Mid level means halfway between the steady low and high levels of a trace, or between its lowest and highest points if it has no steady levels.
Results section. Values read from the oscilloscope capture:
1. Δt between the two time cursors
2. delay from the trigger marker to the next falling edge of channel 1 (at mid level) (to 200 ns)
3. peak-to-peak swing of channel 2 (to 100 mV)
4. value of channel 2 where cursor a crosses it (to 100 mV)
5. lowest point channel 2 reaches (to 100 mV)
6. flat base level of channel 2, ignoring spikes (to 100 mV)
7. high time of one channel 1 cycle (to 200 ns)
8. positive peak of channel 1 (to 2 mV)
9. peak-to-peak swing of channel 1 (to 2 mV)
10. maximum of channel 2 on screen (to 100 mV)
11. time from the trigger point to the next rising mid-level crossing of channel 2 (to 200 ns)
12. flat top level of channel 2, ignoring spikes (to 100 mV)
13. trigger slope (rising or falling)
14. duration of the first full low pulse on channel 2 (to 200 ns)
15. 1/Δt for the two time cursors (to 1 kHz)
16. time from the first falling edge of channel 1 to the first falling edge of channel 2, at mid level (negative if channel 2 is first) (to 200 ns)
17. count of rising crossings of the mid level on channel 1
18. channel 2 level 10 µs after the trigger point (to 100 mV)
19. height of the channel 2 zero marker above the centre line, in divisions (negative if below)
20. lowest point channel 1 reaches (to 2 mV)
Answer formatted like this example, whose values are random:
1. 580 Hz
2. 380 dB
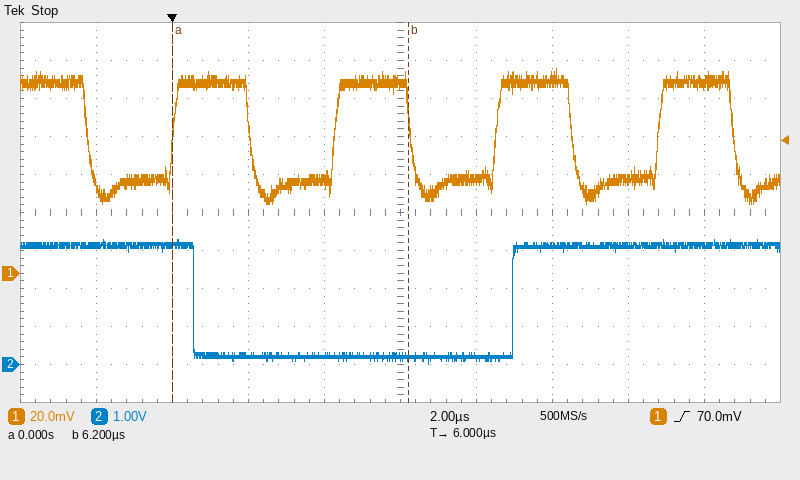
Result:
1. 6.2 µs
2. 2.0 µs
3. 3.3 V
4. 3.1 V
5. 0.0 V
6. 200 mV
7. 2.0 µs
8. 108 mV
9. 72 mV
10. 3.3 V
11. 9.0 µs
12. 3.1 V
13. rising
14. 8.4 µs
15. 161 kHz
16. +2.8 µs
17. 4
18. 3.1 V
19. -4.0 div
20. 36 mV
